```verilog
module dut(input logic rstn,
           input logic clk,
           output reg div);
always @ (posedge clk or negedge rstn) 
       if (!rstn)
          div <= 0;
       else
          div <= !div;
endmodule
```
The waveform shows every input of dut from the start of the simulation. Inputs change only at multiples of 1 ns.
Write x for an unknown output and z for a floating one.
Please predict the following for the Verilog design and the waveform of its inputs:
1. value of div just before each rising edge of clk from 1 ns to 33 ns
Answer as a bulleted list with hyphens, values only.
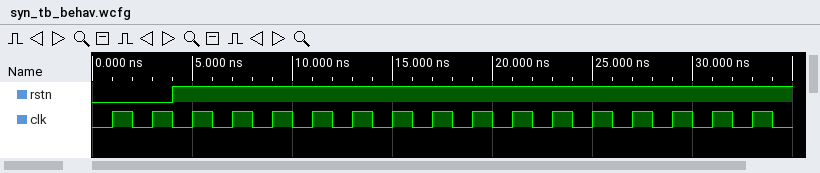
- 0 0 0 1 0 1 0 1 0 1 0 1 0 1 0 1 0
